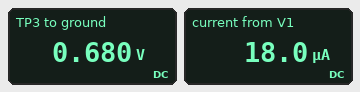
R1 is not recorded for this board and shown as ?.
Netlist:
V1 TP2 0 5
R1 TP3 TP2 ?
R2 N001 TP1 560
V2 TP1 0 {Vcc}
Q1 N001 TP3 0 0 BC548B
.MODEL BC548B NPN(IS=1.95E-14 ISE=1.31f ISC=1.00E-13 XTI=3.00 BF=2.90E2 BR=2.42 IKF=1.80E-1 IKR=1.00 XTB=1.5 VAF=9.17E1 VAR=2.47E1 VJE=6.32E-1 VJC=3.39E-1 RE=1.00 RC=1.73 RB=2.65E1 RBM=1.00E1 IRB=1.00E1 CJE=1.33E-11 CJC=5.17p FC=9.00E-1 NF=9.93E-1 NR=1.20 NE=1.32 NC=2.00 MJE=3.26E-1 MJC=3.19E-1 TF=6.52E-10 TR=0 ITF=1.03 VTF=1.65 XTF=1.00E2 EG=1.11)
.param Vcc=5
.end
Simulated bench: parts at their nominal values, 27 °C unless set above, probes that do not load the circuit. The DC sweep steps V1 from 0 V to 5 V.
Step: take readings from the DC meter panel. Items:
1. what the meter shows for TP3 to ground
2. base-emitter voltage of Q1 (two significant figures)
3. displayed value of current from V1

0.680 V
680 mV
18.0 µA
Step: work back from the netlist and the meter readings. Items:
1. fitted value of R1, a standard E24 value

240 kΩ
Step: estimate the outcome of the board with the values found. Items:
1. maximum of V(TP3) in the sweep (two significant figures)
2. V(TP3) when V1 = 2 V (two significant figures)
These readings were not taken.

680 mV
650 mV
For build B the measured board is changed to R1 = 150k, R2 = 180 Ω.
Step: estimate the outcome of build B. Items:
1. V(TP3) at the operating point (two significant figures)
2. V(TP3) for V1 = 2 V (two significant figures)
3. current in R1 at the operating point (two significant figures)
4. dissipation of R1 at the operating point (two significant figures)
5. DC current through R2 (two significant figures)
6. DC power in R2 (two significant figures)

700 mV
660 mV
29 µA
120 µW
7.8 mA
11 mW
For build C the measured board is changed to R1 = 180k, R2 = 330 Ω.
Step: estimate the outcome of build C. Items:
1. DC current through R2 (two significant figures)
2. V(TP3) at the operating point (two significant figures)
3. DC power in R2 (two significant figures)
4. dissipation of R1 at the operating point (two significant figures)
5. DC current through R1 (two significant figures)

6.5 mA
690 mV
14 mW
100 µW
24 µA
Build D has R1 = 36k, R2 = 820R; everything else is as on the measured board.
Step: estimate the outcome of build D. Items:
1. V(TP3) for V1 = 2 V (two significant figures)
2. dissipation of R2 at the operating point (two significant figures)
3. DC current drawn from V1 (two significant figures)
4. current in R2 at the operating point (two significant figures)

690 mV
31 mW
120 µA
6.1 mA
